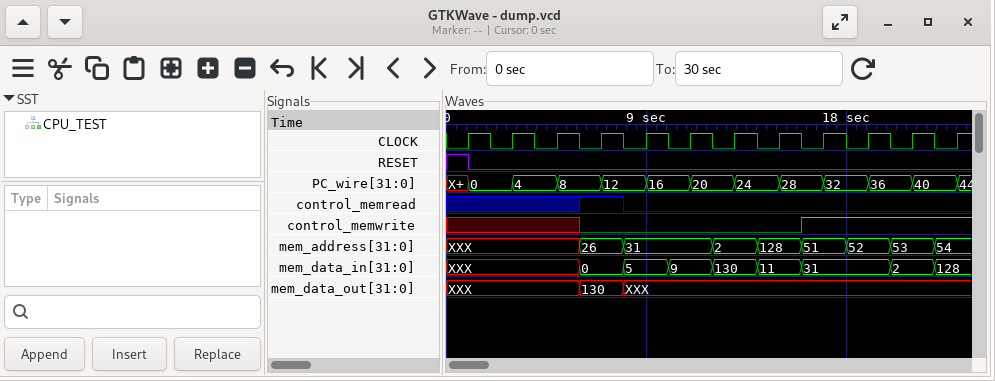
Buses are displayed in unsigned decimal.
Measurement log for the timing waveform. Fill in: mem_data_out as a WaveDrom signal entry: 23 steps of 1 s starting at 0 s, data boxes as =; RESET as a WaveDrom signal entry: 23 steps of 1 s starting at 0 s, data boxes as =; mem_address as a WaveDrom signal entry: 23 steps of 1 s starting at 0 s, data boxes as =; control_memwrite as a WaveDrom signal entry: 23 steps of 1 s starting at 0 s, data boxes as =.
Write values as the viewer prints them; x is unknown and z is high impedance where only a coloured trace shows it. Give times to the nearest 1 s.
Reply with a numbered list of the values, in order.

1. {name: 'mem_data_out', wave: 'x.....=.x..............', data: '130'}
2. {name: 'RESET', wave: '10.....................'}
3. {name: 'mem_address', wave: 'x.....=.=...=.=.=.=.=.=', data: '26 31 2 128 51 52 53 54'}
4. {name: 'control_memwrite', wave: 'x.....0.........1......'}
